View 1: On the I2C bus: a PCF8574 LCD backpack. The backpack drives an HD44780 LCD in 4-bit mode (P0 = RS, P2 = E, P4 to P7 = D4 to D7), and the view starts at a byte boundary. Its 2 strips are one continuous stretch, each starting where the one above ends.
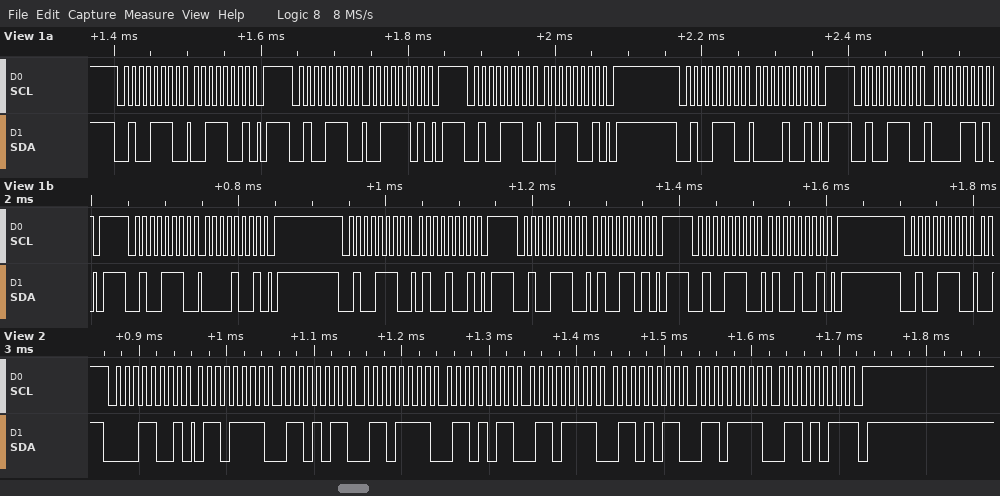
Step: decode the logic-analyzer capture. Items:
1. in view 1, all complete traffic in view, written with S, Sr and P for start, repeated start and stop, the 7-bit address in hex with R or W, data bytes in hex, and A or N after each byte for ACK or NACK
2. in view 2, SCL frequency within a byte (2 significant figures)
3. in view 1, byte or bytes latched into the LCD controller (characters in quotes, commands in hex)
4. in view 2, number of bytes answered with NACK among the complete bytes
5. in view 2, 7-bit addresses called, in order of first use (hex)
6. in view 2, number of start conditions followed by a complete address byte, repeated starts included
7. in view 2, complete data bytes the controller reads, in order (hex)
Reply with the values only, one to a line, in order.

S 27W A 39 A P S 27W A 3D A P S 27W A 39 A P S 27W A 09 A P S 27W A 0D A P S 27W A 09 A P S 27W A 49 A P S 27W A 4D A P S 27W A 49 A P S 27W A
100 kHz
'0'
1
0x0C
1
6F 6B 6F 6B 6F 6B 6F 6B
